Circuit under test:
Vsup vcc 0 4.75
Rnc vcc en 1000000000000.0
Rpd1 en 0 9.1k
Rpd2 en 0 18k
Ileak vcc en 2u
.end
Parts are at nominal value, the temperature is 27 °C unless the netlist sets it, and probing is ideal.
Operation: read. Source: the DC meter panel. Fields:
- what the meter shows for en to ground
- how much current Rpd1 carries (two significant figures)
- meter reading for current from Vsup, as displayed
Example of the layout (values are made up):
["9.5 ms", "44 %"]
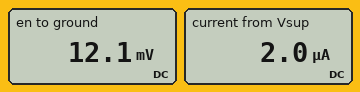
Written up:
["12.1 mV", "1.3 µA", "2.0 µA"]
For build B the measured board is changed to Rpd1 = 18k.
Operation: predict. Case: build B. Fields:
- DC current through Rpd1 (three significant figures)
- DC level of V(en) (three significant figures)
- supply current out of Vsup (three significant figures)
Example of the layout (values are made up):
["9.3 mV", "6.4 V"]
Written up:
["1.00 µA", "18.0 mV", "2.00 µA"]
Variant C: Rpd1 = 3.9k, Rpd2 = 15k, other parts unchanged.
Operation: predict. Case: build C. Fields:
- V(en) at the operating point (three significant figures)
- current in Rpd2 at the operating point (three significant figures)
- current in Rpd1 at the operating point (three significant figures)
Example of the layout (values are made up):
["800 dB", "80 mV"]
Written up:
["6.19 mV", "413 nA", "1.59 µA"]
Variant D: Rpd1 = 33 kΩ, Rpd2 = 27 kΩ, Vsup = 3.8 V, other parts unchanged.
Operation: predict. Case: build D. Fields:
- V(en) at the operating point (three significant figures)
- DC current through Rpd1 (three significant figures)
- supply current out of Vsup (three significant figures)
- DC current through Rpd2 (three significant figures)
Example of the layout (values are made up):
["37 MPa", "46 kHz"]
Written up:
["29.7 mV", "900 nA", "2.00 µA", "1.10 µA"]
